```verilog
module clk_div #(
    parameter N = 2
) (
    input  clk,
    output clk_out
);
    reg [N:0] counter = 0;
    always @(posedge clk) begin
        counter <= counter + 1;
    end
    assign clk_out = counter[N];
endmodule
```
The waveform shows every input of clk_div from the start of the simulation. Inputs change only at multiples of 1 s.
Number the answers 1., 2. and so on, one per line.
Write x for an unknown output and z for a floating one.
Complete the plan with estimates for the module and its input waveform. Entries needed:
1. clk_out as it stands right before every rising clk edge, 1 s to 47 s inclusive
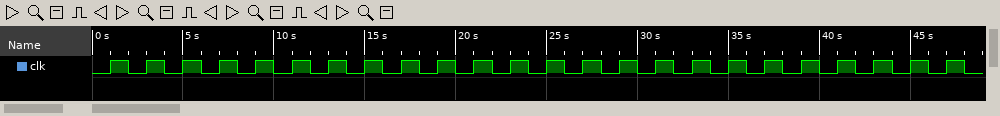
1. 0 0 0 0 1 1 1 1 0 0 0 0 1 1 1 1 0 0 0 0 1 1 1 1
